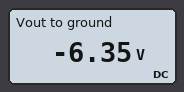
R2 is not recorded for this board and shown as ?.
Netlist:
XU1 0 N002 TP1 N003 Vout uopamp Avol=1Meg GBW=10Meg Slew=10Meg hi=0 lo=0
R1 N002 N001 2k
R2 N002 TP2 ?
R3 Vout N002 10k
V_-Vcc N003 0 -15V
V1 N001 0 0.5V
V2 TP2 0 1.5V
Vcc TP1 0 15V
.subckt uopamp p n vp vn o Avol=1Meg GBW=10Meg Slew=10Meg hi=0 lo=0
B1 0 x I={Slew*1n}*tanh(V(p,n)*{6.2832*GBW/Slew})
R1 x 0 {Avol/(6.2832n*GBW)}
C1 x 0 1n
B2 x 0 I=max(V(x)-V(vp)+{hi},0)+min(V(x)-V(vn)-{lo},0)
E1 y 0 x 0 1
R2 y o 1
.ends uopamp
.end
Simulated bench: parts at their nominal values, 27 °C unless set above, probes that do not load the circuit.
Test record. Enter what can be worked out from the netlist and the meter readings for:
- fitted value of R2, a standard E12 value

3.9 kΩ
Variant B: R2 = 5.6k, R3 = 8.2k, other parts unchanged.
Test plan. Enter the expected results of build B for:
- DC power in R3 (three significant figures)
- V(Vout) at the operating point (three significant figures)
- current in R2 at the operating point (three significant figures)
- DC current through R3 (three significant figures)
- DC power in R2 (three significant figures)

2.20 mW
-4.25 V
268 µA
518 µA
402 µW
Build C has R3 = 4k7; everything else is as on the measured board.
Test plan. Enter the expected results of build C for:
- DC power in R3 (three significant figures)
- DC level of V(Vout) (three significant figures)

1.89 mW
-2.98 V
